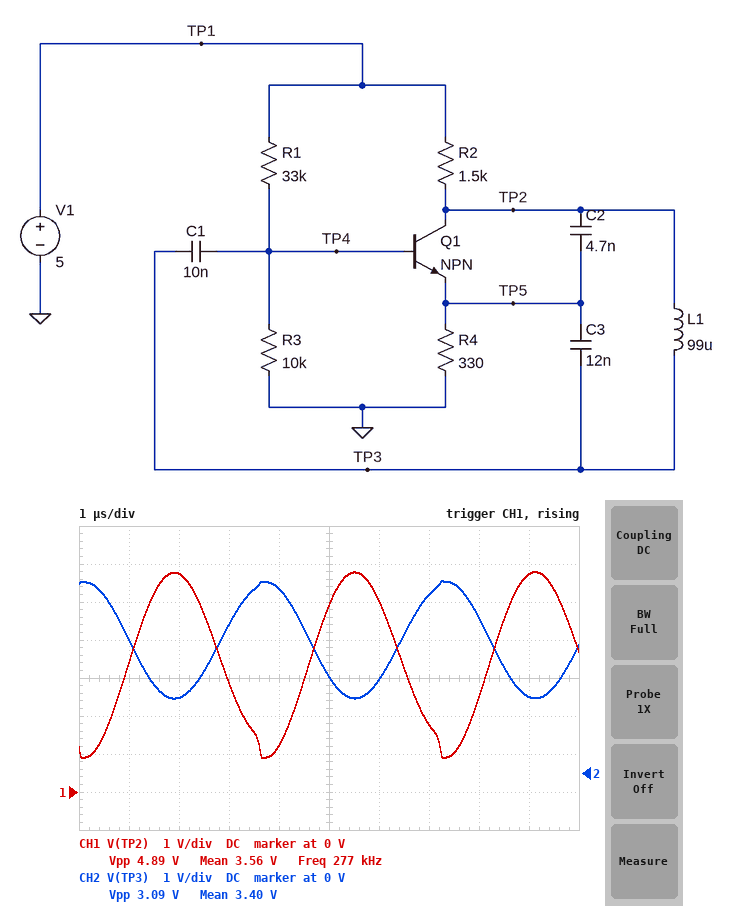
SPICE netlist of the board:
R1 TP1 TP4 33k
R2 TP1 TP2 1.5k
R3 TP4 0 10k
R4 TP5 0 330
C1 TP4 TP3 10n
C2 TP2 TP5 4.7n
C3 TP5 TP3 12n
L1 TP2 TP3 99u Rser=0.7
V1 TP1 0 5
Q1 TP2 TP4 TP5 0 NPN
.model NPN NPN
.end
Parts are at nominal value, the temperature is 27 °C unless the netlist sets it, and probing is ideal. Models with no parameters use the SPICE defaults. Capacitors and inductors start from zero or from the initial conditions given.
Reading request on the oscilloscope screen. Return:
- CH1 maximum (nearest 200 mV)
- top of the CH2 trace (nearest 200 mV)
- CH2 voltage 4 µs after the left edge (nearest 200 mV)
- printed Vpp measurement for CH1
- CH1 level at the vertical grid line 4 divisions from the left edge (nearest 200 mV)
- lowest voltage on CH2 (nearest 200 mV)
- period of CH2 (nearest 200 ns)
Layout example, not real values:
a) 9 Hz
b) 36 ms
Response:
a) 5.8 V
b) 5.0 V
c) 4.8 V
d) 4.89 V
e) 1.2 V
f) 2.0 V
g) 3.6 µs
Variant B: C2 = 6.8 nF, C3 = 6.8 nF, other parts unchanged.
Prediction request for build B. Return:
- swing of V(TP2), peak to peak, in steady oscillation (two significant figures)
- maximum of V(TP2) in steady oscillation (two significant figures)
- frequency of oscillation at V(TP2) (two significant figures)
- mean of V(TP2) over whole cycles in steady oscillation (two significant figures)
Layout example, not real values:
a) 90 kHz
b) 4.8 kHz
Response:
a) 4.0 V
b) 4.9 V
c) 280 kHz
d) 3.0 V
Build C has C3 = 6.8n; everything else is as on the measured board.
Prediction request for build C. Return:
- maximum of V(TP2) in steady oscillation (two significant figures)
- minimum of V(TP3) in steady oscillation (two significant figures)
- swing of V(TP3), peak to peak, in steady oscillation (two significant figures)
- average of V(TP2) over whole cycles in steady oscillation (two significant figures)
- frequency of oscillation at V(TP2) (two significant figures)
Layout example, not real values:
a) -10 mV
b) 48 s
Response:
a) 5.4 V
b) 1.2 V
c) 4.2 V
d) 3.3 V
e) 310 kHz
